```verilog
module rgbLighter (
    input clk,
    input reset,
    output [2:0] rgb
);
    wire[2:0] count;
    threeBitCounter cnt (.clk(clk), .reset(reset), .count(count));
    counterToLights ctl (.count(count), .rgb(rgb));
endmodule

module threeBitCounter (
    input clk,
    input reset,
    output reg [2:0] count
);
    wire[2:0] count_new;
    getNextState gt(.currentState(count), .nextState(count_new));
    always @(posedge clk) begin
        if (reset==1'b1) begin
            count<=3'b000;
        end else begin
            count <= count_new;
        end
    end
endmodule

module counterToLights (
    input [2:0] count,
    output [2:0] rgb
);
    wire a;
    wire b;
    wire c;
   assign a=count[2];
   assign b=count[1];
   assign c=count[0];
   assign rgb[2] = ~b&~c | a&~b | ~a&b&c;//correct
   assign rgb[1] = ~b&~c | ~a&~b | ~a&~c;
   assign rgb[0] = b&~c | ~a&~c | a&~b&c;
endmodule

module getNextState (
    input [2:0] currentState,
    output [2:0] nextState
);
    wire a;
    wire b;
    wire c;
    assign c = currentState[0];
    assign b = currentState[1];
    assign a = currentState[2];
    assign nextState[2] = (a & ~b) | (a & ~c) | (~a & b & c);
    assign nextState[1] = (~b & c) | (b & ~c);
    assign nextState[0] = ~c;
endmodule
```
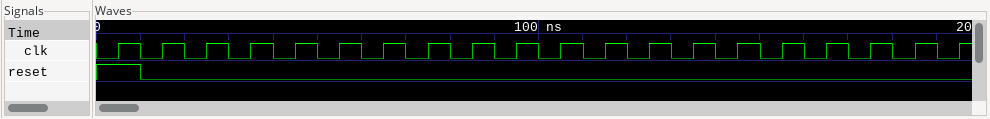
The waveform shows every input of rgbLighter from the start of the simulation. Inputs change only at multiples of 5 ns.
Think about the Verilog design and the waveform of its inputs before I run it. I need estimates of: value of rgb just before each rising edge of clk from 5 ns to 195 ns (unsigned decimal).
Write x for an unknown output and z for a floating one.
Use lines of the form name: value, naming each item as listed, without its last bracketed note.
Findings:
value of rgb just before each rising edge of clk from 5 ns to 195 ns: x, 7, 2, 3, 4, 6, 5, 1, 0, 7, 2, 3, 4, 6, 5, 1, 0, 7, 2, 3
